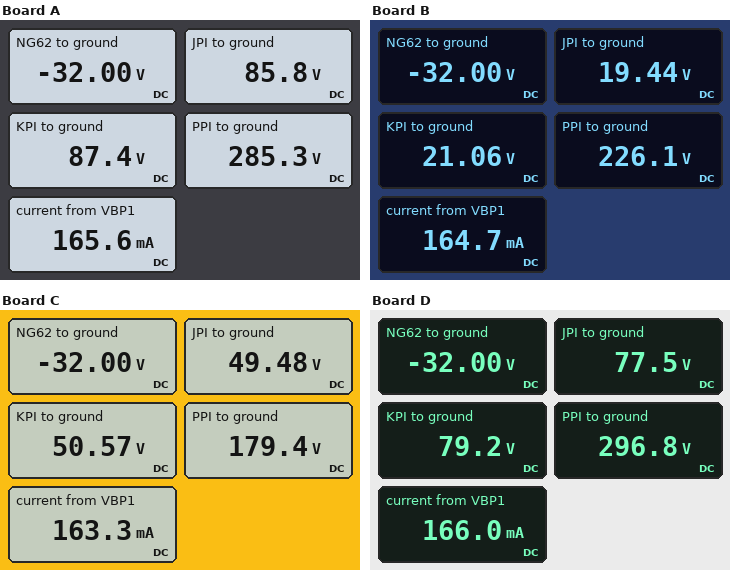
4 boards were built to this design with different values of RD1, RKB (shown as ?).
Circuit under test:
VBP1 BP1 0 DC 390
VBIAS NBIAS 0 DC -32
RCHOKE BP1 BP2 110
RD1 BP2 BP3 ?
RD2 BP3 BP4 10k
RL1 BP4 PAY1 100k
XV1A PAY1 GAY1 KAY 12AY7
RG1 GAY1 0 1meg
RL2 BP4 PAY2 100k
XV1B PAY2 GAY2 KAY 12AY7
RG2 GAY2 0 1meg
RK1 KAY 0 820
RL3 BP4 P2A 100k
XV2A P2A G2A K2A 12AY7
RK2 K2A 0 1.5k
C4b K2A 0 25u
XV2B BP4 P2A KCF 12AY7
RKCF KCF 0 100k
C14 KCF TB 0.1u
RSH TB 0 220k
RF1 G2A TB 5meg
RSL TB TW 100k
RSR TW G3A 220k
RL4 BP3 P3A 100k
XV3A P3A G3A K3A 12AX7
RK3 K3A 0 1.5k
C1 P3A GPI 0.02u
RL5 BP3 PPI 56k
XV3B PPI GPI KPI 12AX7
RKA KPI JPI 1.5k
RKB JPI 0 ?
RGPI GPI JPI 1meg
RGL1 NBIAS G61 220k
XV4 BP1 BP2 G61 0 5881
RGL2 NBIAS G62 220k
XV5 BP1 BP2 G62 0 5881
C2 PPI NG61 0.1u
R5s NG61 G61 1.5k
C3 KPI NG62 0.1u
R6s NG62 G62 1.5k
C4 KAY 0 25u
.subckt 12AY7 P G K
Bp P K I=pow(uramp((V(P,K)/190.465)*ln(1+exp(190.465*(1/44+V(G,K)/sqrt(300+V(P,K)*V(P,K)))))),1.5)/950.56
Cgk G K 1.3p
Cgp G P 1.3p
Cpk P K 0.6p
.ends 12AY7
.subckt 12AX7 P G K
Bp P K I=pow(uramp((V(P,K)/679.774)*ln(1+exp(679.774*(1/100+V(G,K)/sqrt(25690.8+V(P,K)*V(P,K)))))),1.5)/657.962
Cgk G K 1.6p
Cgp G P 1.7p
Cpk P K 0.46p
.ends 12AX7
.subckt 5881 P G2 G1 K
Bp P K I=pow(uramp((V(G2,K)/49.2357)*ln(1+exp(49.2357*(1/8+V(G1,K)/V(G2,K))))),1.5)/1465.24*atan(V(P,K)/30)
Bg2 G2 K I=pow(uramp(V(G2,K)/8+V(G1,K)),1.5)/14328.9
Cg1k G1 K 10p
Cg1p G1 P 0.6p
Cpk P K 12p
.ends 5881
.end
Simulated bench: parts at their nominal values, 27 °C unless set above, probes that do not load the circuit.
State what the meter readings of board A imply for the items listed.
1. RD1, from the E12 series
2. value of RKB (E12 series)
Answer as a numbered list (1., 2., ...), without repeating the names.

1. 5.6 kΩ
2. 82 kΩ
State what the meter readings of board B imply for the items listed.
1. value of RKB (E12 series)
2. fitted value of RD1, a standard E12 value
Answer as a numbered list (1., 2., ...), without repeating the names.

1. 18 kΩ
2. 15 kΩ
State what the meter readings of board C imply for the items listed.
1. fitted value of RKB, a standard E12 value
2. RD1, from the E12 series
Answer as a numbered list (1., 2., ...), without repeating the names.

1. 68 kΩ
2. 33 kΩ
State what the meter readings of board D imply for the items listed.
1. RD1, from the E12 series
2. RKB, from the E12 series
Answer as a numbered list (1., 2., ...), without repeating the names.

1. 3.3 kΩ
2. 68 kΩ
